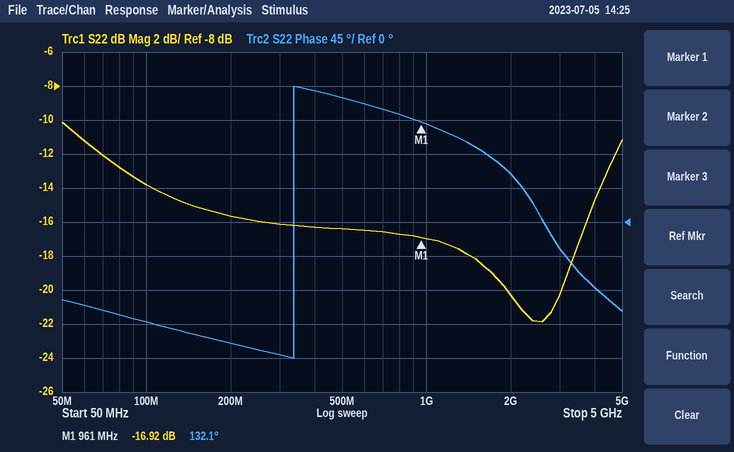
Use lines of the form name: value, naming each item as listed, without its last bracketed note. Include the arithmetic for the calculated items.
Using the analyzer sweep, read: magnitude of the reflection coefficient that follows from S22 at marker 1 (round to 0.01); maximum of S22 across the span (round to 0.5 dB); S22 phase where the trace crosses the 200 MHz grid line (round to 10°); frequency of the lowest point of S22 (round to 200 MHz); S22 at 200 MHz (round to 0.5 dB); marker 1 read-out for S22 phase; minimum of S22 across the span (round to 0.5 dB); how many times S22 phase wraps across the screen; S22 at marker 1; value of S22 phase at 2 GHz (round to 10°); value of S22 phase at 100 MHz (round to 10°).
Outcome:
magnitude of the reflection coefficient that follows from S22 at marker 1: 10^(-16.92/20) ≈ 0.14
maximum of S22 across the span: -10.0 dB
S22 phase where the trace crosses the 200 MHz grid line: -160°
frequency of the lowest point of S22: 2.6 GHz
S22 at 200 MHz: -15.5 dB
marker 1 read-out for S22 phase: 132.1°
minimum of S22 across the span: -22.0 dB
how many times S22 phase wraps across the screen: 1
S22 at marker 1: -16.92 dB
value of S22 phase at 2 GHz: 60°
value of S22 phase at 100 MHz: -130°
